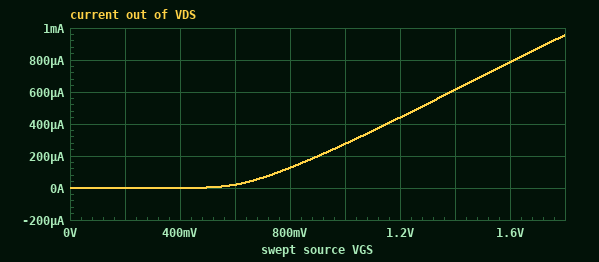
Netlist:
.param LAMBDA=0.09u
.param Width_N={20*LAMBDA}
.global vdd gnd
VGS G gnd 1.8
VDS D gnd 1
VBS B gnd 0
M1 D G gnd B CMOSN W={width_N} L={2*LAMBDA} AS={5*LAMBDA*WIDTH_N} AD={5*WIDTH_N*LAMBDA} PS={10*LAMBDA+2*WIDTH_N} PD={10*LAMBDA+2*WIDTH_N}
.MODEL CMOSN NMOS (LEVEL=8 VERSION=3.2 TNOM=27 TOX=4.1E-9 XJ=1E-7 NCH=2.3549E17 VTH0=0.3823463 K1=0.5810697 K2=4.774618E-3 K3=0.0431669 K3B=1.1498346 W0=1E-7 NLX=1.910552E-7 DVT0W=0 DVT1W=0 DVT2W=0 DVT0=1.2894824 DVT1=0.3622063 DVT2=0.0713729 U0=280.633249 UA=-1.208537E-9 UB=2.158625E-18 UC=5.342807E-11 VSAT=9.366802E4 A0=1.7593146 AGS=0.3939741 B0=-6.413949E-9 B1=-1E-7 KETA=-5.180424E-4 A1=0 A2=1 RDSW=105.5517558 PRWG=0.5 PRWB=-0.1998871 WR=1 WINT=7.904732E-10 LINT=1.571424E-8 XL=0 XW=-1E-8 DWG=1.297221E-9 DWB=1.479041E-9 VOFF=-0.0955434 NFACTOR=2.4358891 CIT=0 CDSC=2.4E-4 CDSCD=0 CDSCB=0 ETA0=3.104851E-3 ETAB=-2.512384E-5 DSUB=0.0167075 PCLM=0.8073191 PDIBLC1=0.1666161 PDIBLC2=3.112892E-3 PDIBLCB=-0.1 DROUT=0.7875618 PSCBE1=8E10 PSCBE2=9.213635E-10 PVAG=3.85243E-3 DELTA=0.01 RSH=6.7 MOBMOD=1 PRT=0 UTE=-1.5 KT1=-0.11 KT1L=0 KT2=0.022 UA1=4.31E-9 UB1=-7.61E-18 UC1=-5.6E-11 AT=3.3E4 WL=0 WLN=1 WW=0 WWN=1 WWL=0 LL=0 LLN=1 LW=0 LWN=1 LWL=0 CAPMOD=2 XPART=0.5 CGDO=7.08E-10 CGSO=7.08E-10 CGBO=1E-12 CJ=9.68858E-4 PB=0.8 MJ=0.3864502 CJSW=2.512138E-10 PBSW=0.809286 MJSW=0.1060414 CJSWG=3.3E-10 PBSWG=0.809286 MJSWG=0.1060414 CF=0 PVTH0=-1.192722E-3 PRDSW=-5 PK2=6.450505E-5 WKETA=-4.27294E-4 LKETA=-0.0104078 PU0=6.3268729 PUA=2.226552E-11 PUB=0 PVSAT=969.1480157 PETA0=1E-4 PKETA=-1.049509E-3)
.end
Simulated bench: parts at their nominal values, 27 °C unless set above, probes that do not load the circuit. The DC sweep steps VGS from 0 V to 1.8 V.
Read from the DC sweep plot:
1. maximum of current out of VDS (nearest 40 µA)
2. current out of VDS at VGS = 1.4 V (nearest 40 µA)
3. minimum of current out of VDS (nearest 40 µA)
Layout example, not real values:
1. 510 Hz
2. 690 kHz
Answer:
1. 960 µA
2. 600 µA
3. 0 A
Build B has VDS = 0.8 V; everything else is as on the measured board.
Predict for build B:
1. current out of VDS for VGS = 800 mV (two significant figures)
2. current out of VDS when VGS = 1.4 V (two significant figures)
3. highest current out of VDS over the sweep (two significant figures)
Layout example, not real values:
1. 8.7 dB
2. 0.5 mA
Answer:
1. 120 µA
2. 600 µA
3. 930 µA
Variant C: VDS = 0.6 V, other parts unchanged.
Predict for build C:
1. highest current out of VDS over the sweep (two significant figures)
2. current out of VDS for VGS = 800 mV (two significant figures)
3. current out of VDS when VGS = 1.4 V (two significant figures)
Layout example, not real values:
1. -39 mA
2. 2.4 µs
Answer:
1. 880 µA
2. 120 µA
3. 580 µA
